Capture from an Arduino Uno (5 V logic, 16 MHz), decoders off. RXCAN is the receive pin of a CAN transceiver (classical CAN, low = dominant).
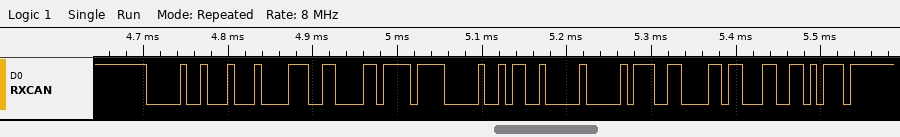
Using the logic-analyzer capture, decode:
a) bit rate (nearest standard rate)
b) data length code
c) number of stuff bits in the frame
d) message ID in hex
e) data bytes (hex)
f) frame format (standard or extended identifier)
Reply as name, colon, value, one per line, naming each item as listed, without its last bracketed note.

bit rate: 125 kbit/s
data length code: 8
number of stuff bits in the frame: 4
message ID in hex: 0x011
data bytes: 73 0D EF 01 64 00 73 0D
frame format: standard
